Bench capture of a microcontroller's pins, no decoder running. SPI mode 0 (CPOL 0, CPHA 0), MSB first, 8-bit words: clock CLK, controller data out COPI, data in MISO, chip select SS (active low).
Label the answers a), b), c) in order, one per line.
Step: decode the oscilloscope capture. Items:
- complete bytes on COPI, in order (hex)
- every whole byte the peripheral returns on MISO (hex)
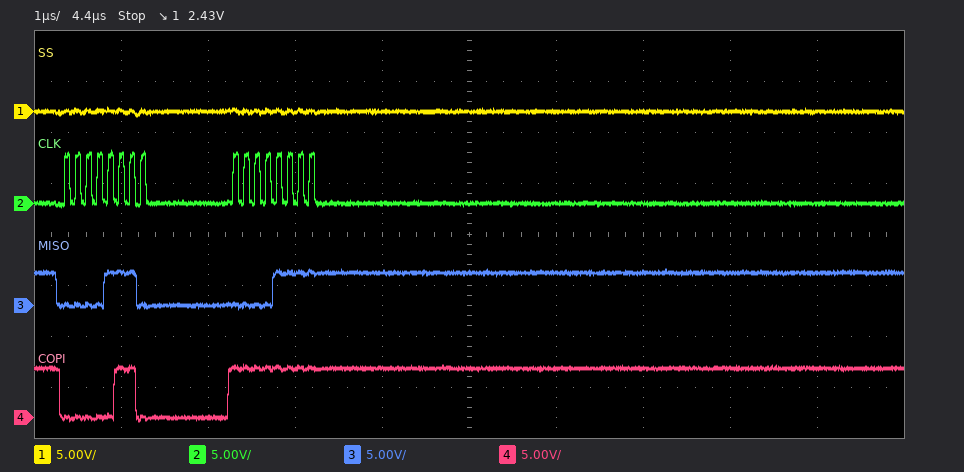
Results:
a) 06 FF
b) 0E 0F
